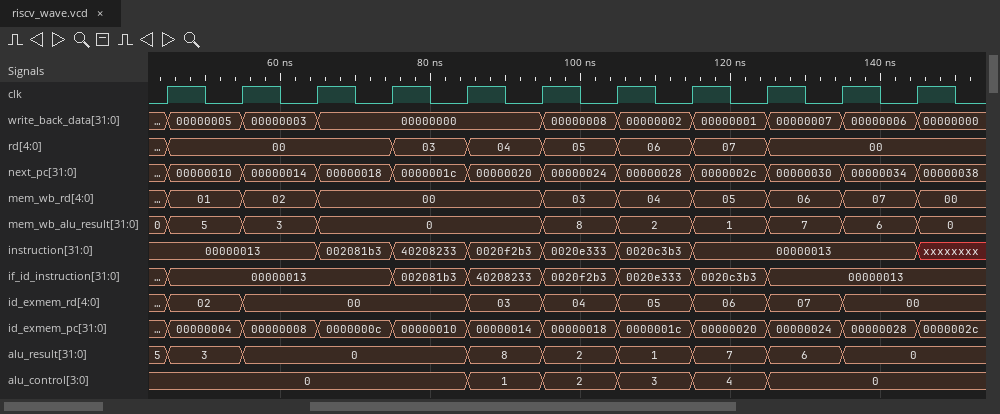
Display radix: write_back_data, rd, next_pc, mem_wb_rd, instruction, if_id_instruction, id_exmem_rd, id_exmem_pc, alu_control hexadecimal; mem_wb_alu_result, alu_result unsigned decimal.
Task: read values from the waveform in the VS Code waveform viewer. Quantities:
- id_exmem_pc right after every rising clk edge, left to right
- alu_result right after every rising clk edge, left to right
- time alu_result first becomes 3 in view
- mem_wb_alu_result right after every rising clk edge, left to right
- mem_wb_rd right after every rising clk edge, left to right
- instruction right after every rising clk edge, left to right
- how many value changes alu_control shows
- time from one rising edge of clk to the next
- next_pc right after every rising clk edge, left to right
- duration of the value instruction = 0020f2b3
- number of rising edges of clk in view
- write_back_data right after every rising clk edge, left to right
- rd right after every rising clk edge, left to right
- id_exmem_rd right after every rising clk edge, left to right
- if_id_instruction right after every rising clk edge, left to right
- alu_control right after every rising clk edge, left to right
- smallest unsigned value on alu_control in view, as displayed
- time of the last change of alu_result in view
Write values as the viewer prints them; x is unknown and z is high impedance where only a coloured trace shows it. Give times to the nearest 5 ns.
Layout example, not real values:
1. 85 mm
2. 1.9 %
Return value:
1. 00000004, 00000008, 0000000c, 00000010, 00000014, 00000018, 0000001c, 00000020, 00000024, 00000028, 0000002c
2. 3, 0, 0, 0, 8, 2, 1, 7, 6, 0, 0
3. 45 ns
4. 5, 3, 0, 0, 0, 8, 2, 1, 7, 6, 0
5. 01, 02, 00, 00, 00, 03, 04, 05, 06, 07, 00
6. 00000013, 00000013, 002081b3, 40208233, 0020f2b3, 0020e333, 0020c3b3, 00000013, 00000013, 00000013, xxxxxxxx
7. 5
8. 10 ns
9. 00000010, 00000014, 00000018, 0000001c, 00000020, 00000024, 00000028, 0000002c, 00000030, 00000034, 00000038
10. 10 ns
11. 11
12. 00000005, 00000003, 00000000, 00000000, 00000000, 00000008, 00000002, 00000001, 00000007, 00000006, 00000000
13. 00, 00, 00, 03, 04, 05, 06, 07, 00, 00, 00
14. 02, 00, 00, 00, 03, 04, 05, 06, 07, 00, 00
15. 00000013, 00000013, 00000013, 002081b3, 40208233, 0020f2b3, 0020e333, 0020c3b3, 00000013, 00000013, 00000013
16. 0, 0, 0, 0, 1, 2, 3, 4, 0, 0, 0
17. 0
18. 135 ns
